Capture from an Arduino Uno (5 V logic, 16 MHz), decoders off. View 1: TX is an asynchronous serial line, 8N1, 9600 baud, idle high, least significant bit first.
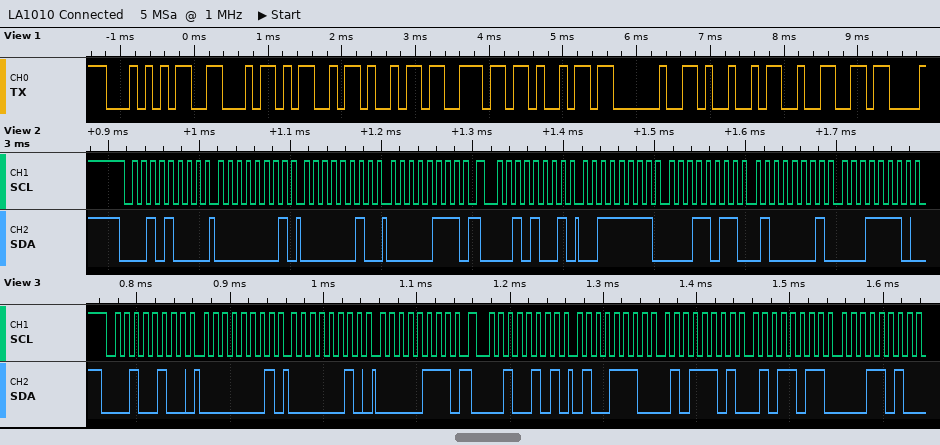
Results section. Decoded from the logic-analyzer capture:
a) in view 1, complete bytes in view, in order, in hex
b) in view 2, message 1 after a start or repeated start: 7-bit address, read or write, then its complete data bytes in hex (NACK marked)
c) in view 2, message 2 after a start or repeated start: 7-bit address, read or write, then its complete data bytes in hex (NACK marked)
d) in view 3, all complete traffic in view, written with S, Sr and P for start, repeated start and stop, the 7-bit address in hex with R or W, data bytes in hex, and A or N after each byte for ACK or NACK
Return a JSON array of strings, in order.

["0x54 0x46 0x4D 0x69 0x6E 0x69 0x20 0x49 0x32", "0x14 write: 01 02 07", "0x14 read: 3F 1B 41 1E", "S 12W A 01 A 02 A 07 A Sr 12R A 4E A 5D A 5B A 1A A"]
